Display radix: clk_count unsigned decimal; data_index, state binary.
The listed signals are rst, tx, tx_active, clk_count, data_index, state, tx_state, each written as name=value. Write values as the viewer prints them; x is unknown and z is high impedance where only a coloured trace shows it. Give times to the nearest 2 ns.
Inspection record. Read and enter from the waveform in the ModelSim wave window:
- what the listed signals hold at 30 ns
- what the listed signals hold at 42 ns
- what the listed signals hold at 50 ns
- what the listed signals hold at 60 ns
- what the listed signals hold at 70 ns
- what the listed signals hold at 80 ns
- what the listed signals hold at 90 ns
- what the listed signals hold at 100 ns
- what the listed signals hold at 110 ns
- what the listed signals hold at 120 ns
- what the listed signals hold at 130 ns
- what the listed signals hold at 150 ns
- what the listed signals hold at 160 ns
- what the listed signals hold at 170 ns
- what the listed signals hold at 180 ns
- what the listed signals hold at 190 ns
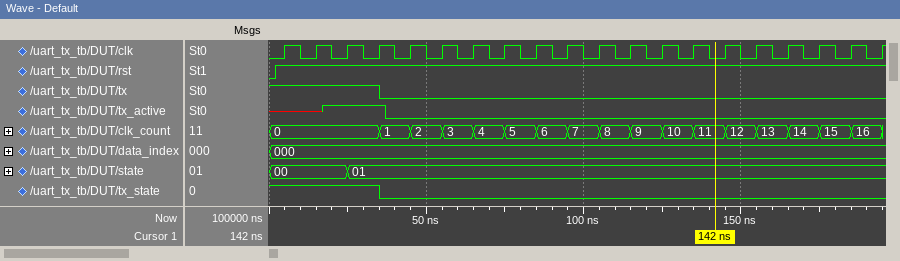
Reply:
rst=1, tx=1, tx_active=1, clk_count=0, data_index=000, state=01, tx_state=1
rst=1, tx=0, tx_active=0, clk_count=1, data_index=000, state=01, tx_state=0
rst=1, tx=0, tx_active=0, clk_count=2, data_index=000, state=01, tx_state=0
rst=1, tx=0, tx_active=0, clk_count=3, data_index=000, state=01, tx_state=0
rst=1, tx=0, tx_active=0, clk_count=4, data_index=000, state=01, tx_state=0
rst=1, tx=0, tx_active=0, clk_count=5, data_index=000, state=01, tx_state=0
rst=1, tx=0, tx_active=0, clk_count=6, data_index=000, state=01, tx_state=0
rst=1, tx=0, tx_active=0, clk_count=7, data_index=000, state=01, tx_state=0
rst=1, tx=0, tx_active=0, clk_count=8, data_index=000, state=01, tx_state=0
rst=1, tx=0, tx_active=0, clk_count=9, data_index=000, state=01, tx_state=0
rst=1, tx=0, tx_active=0, clk_count=10, data_index=000, state=01, tx_state=0
rst=1, tx=0, tx_active=0, clk_count=12, data_index=000, state=01, tx_state=0
rst=1, tx=0, tx_active=0, clk_count=13, data_index=000, state=01, tx_state=0
rst=1, tx=0, tx_active=0, clk_count=14, data_index=000, state=01, tx_state=0
rst=1, tx=0, tx_active=0, clk_count=15, data_index=000, state=01, tx_state=0
rst=1, tx=0, tx_active=0, clk_count=16, data_index=000, state=01, tx_state=0
